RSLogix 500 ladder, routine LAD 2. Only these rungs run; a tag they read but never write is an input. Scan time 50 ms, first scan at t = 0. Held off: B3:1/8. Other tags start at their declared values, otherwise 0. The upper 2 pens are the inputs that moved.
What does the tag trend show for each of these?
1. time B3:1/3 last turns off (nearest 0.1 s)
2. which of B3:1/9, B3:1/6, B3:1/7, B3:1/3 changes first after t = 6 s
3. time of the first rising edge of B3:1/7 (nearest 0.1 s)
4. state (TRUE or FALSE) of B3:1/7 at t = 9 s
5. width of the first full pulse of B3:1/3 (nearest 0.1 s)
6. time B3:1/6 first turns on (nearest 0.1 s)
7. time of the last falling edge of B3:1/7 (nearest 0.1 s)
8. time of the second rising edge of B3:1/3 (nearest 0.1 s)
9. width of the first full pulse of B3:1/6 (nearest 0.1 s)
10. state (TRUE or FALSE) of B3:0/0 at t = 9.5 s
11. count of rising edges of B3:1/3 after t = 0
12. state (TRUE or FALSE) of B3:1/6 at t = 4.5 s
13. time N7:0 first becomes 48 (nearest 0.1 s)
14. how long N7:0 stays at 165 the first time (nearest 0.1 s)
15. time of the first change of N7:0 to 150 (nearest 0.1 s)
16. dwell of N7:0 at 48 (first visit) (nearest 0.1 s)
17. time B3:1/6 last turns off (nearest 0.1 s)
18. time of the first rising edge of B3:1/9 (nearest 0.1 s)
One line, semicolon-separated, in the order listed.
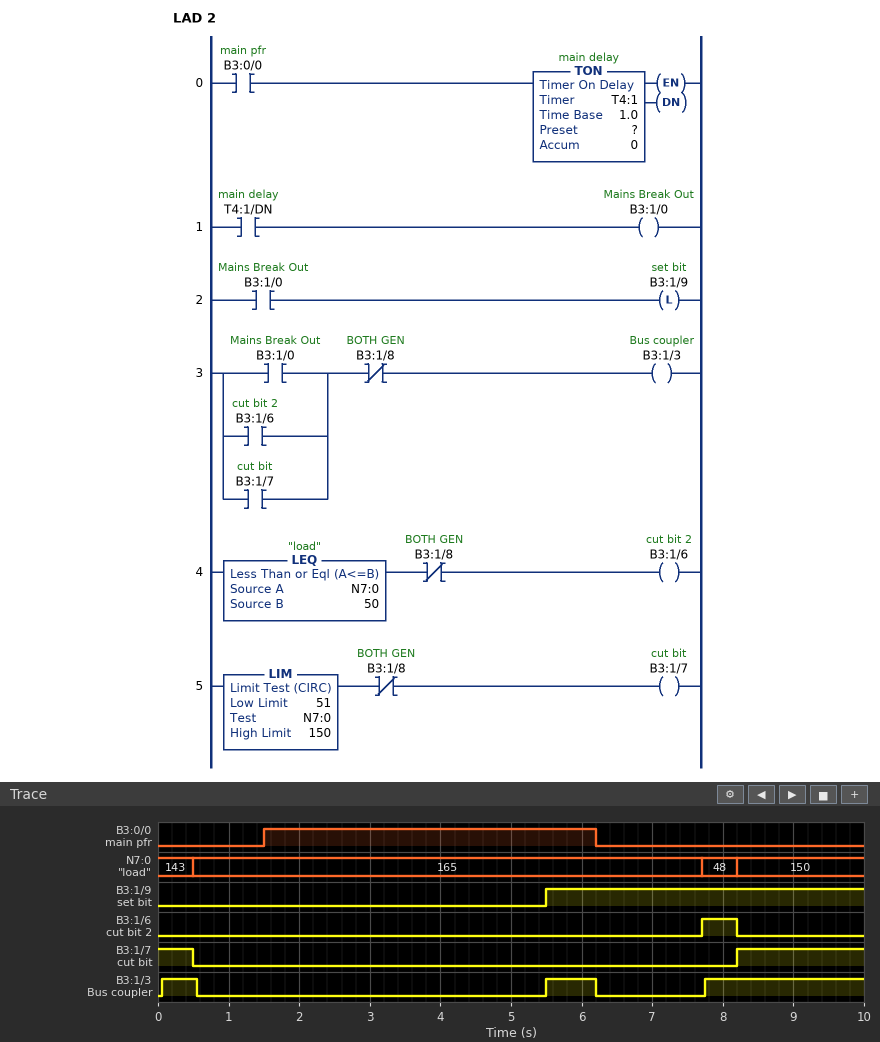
6.2 s; B3:1/3; 8.2 s; TRUE; 0.5 s; 7.7 s; 0.5 s; 5.5 s; 0.5 s; FALSE; 3; FALSE; 7.7 s; 7.2 s; 8.2 s; 0.5 s; 8.2 s; 5.5 s
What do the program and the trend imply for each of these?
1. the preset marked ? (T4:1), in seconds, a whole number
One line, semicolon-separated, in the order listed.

4 s
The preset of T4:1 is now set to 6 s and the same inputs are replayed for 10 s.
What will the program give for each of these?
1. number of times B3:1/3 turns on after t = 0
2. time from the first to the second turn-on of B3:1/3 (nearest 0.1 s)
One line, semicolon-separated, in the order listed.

2; 7.7 s
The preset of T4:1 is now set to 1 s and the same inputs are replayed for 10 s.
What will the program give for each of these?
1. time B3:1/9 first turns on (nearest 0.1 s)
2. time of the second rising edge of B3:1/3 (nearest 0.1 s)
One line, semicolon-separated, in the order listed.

2.5 s; 2.5 s
